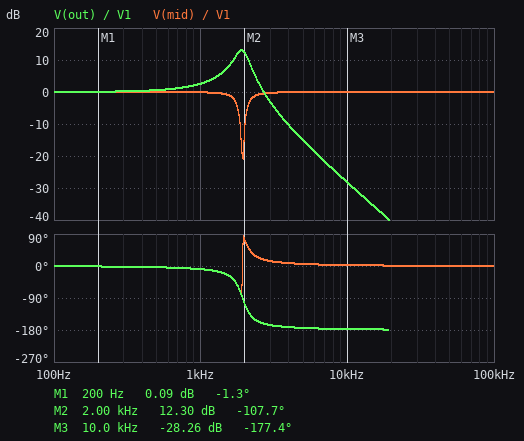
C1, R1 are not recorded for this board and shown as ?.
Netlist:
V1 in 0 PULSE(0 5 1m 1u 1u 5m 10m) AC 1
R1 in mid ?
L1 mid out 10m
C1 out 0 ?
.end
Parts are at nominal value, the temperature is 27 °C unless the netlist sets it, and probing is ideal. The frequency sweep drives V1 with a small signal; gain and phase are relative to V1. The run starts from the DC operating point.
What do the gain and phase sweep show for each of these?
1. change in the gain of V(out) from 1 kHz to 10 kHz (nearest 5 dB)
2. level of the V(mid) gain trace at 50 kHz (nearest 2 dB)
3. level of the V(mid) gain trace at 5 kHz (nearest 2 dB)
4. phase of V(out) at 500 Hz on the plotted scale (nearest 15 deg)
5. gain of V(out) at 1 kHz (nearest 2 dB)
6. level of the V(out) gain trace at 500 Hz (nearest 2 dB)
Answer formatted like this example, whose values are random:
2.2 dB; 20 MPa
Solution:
-30 dB; 0 dB; 0 dB; 0 deg; 2 dB; 0 dB
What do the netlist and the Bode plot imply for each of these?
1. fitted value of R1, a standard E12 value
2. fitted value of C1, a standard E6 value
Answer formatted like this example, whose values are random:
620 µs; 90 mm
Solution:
27 Ω; 680 nF
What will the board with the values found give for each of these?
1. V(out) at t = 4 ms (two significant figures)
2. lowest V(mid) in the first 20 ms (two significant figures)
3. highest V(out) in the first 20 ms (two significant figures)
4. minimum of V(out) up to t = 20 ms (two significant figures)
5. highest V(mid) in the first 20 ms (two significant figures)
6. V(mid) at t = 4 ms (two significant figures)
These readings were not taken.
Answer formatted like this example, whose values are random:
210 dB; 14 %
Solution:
5.0 V; -670 mV; 8.5 V; -3.5 V; 5.7 V; 5.0 V
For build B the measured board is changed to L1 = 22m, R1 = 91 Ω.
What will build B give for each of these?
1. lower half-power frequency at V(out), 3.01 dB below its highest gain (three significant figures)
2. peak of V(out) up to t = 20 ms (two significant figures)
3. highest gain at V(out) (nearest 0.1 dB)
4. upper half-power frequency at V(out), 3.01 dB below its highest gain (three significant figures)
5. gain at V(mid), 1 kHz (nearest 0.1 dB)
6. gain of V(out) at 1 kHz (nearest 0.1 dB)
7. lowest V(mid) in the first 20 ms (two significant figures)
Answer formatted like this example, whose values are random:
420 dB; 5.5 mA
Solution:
805 Hz; 7.2 V; 6.2 dB; 1.52 kHz; -2.8 dB; 5.0 dB; -790 mV
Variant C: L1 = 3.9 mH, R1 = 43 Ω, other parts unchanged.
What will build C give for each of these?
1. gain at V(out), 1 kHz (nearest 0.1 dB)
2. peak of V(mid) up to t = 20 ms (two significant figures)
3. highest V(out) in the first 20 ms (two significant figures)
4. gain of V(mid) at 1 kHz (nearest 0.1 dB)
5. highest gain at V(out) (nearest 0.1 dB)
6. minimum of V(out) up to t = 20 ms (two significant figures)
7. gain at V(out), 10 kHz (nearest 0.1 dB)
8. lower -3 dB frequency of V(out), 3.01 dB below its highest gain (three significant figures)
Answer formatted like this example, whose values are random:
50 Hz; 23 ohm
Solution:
0.8 dB; 5.8 V; 7.0 V; -0.2 dB; 5.3 dB; -2.0 V; -19.7 dB; 1.68 kHz
